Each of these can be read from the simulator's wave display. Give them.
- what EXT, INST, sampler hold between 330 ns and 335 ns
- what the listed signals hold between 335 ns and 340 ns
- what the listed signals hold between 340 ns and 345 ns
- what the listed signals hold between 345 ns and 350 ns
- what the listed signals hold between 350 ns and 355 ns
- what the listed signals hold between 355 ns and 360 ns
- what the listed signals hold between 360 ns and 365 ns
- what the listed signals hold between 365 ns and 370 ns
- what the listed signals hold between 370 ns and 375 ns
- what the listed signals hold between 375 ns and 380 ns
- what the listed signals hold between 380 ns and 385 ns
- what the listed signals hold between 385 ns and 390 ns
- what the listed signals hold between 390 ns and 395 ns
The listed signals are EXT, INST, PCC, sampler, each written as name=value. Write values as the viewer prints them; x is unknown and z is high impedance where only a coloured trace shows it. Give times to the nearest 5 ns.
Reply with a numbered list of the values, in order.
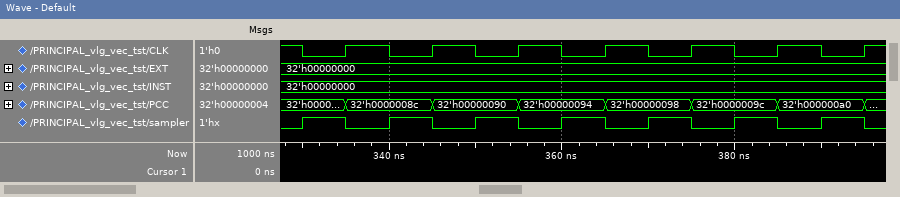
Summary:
1. EXT=32'h00000000, INST=32'h00000000, sampler=1
2. EXT=32'h00000000, INST=32'h00000000, PCC=32'h0000008c, sampler=0
3. EXT=32'h00000000, INST=32'h00000000, PCC=32'h0000008c, sampler=1
4. EXT=32'h00000000, INST=32'h00000000, PCC=32'h00000090, sampler=0
5. EXT=32'h00000000, INST=32'h00000000, PCC=32'h00000090, sampler=1
6. EXT=32'h00000000, INST=32'h00000000, PCC=32'h00000094, sampler=0
7. EXT=32'h00000000, INST=32'h00000000, PCC=32'h00000094, sampler=1
8. EXT=32'h00000000, INST=32'h00000000, PCC=32'h00000098, sampler=0
9. EXT=32'h00000000, INST=32'h00000000, PCC=32'h00000098, sampler=1
10. EXT=32'h00000000, INST=32'h00000000, PCC=32'h0000009c, sampler=0
11. EXT=32'h00000000, INST=32'h00000000, PCC=32'h0000009c, sampler=1
12. EXT=32'h00000000, INST=32'h00000000, PCC=32'h000000a0, sampler=0
13. EXT=32'h00000000, INST=32'h00000000, PCC=32'h000000a0, sampler=1
